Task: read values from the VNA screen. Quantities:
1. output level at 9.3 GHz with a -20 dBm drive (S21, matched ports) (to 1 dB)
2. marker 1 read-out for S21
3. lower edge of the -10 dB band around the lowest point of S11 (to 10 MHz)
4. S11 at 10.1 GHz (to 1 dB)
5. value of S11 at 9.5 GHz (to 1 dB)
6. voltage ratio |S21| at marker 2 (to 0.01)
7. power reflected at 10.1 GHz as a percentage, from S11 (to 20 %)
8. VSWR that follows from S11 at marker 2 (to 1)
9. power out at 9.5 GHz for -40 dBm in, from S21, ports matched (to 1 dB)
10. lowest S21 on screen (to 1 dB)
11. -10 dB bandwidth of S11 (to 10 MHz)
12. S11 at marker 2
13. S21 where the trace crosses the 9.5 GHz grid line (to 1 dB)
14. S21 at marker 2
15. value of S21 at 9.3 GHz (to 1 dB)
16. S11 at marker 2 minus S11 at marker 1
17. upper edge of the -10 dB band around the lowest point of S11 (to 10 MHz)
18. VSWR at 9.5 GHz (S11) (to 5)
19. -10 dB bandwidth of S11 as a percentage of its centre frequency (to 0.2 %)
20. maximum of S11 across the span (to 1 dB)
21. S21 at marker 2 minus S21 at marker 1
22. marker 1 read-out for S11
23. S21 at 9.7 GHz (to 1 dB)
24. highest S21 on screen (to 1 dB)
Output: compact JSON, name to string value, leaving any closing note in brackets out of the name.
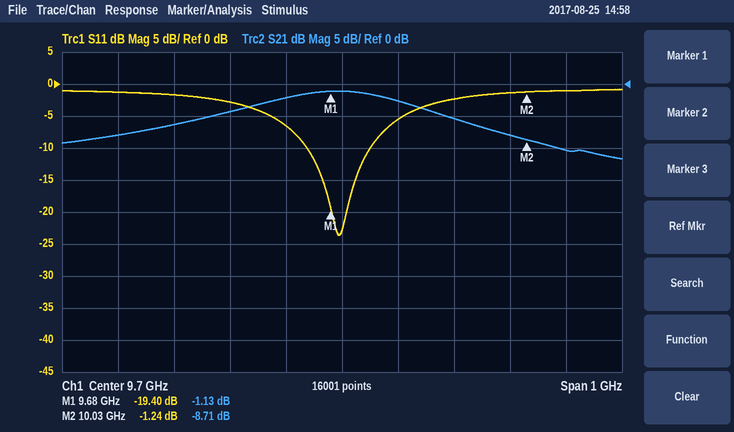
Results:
{"output level at 9.3 GHz with a -20 dBm drive (S21, matched ports)": "-28 dBm", "marker 1 read-out for S21": "-1.13 dB", "lower edge of the -10 dB band around the lowest point of S11": "9.64 GHz", "S11 at 10.1 GHz": "-1 dB", "value of S11 at 9.5 GHz": "-3 dB", "voltage ratio |S21| at marker 2": "0.37", "power reflected at 10.1 GHz as a percentage, from S11": "80 %", "VSWR that follows from S11 at marker 2": "14", "power out at 9.5 GHz for -40 dBm in, from S21, ports matched": "-44 dBm", "lowest S21 on screen": "-12 dB", "-10 dB bandwidth of S11": "110 MHz", "S11 at marker 2": "-1.24 dB", "S21 where the trace crosses the 9.5 GHz grid line": "-4 dB", "S21 at marker 2": "-8.71 dB", "value of S21 at 9.3 GHz": "-8 dB", "S11 at marker 2 minus S11 at marker 1": "18.16 dB", "upper edge of the -10 dB band around the lowest point of S11": "9.75 GHz", "VSWR at 9.5 GHz (S11)": "5", "-10 dB bandwidth of S11 as a percentage of its centre frequency": "1.2 %", "maximum of S11 across the span": "-1 dB", "S21 at marker 2 minus S21 at marker 1": "-7.58 dB", "marker 1 read-out for S11": "-19.40 dB", "S21 at 9.7 GHz": "-1 dB", "highest S21 on screen": "-1 dB"}
